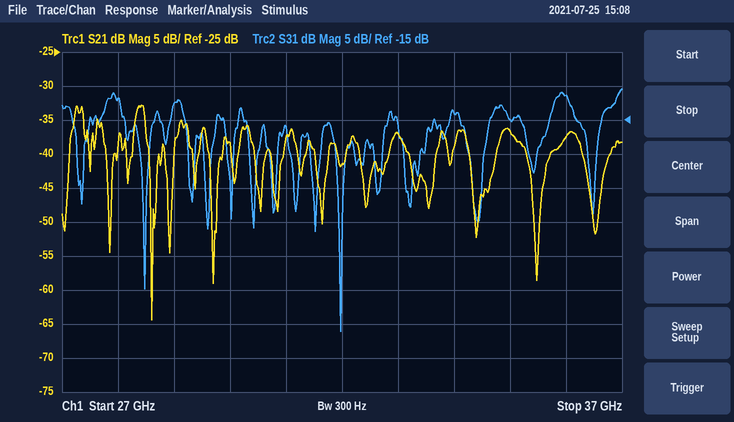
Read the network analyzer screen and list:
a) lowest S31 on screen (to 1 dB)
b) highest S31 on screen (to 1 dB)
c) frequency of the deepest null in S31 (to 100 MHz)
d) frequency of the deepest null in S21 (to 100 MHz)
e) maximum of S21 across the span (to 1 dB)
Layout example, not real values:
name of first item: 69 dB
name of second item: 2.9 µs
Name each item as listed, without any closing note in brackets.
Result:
lowest S31 on screen: -46 dB
highest S31 on screen: -10 dB
frequency of the deepest null in S31: 32.0 GHz
frequency of the deepest null in S21: 28.6 GHz
maximum of S21 across the span: -33 dB
